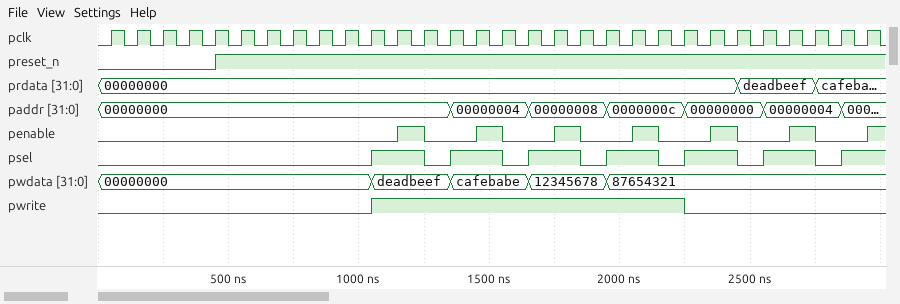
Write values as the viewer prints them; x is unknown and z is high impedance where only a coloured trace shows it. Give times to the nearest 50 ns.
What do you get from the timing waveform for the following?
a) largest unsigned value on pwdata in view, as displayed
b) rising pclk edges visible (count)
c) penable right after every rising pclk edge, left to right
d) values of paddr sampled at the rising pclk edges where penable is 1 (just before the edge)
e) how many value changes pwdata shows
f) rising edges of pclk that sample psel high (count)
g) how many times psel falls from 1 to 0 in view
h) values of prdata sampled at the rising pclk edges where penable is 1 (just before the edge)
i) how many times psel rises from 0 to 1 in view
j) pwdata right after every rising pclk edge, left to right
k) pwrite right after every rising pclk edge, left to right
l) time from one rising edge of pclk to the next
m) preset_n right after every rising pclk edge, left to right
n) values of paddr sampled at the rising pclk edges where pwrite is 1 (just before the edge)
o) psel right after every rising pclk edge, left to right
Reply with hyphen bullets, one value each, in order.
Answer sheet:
- deadbeef
- 30
- 0 0 0 0 0 0 0 0 0 0 0 1 0 0 1 0 0 1 0 0 1 0 0 1 0 0 1 0 0 1
- 00000000, 00000004, 00000008, 0000000c, 00000000, 00000004
- 4
- 13
- 6
- 00000000, 00000000, 00000000, 00000000, 00000000, deadbeef
- 7
- 00000000, 00000000, 00000000, 00000000, 00000000, 00000000, 00000000, 00000000, 00000000, 00000000, deadbeef, deadbeef, deadbeef, cafebabe, cafebabe, cafebabe, 12345678, 12345678, 12345678, 87654321, 87654321, 87654321, 87654321, 87654321, 87654321, 87654321, 87654321, 87654321, 87654321, 87654321
- 0 0 0 0 0 0 0 0 0 0 1 1 1 1 1 1 1 1 1 1 1 1 0 0 0 0 0 0 0 0
- 100 ns
- 0 0 0 0 1 1 1 1 1 1 1 1 1 1 1 1 1 1 1 1 1 1 1 1 1 1 1 1 1 1
- 00000000, 00000000, 00000000, 00000004, 00000004, 00000004, 00000008, 00000008, 00000008, 0000000c, 0000000c, 0000000c
- 0 0 0 0 0 0 0 0 0 0 1 1 0 1 1 0 1 1 0 1 1 0 1 1 0 1 1 0 1 1
